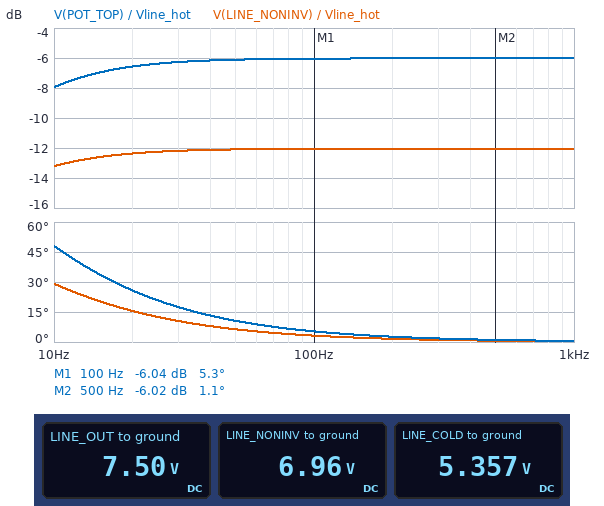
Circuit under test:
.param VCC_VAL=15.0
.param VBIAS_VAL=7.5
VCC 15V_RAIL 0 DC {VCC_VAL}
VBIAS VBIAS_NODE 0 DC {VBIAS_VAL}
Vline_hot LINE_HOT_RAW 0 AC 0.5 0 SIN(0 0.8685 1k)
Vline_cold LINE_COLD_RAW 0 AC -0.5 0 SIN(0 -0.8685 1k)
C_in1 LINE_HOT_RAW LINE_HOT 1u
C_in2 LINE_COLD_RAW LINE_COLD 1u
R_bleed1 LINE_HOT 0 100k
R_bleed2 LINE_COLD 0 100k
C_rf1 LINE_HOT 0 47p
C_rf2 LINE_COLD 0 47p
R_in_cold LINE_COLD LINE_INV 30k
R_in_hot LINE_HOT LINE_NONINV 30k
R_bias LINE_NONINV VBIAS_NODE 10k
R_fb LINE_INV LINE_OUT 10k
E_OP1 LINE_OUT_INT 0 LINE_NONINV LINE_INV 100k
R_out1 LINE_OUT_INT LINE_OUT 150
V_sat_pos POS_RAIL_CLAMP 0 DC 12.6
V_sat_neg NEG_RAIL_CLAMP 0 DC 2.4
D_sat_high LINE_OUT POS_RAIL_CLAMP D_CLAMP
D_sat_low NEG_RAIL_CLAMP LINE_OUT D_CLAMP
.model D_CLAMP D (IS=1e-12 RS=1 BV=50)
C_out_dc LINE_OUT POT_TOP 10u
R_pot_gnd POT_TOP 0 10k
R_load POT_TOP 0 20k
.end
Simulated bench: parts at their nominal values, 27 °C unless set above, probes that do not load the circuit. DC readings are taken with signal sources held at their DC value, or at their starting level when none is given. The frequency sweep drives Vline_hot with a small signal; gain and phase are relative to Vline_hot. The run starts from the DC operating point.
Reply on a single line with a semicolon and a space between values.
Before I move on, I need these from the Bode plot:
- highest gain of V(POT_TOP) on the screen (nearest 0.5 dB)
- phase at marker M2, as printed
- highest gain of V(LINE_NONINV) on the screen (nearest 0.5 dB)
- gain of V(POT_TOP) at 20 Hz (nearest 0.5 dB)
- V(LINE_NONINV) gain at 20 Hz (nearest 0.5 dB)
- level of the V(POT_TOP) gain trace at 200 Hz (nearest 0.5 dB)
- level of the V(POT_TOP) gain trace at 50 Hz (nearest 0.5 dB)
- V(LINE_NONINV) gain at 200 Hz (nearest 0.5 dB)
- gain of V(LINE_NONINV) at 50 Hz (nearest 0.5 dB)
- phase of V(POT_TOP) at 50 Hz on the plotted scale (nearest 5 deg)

-6.0 dB; 1.1 deg; -12.0 dB; -6.5 dB; -12.5 dB; -6.0 dB; -6.0 dB; -12.0 dB; -12.0 dB; 10 deg
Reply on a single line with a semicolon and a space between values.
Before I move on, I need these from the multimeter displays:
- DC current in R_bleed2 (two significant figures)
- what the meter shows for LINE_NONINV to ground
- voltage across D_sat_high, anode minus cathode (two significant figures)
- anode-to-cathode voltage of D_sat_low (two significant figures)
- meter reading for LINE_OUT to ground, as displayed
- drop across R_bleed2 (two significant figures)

54 µA; 6.96 V; -5.1 V; -5.1 V; 7.50 V; 5.4 V
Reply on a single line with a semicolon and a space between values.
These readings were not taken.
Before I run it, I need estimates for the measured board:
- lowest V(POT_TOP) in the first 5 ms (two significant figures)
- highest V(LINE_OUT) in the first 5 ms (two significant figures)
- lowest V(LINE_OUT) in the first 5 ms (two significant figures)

-580 mV; 8.1 V; 6.9 V
